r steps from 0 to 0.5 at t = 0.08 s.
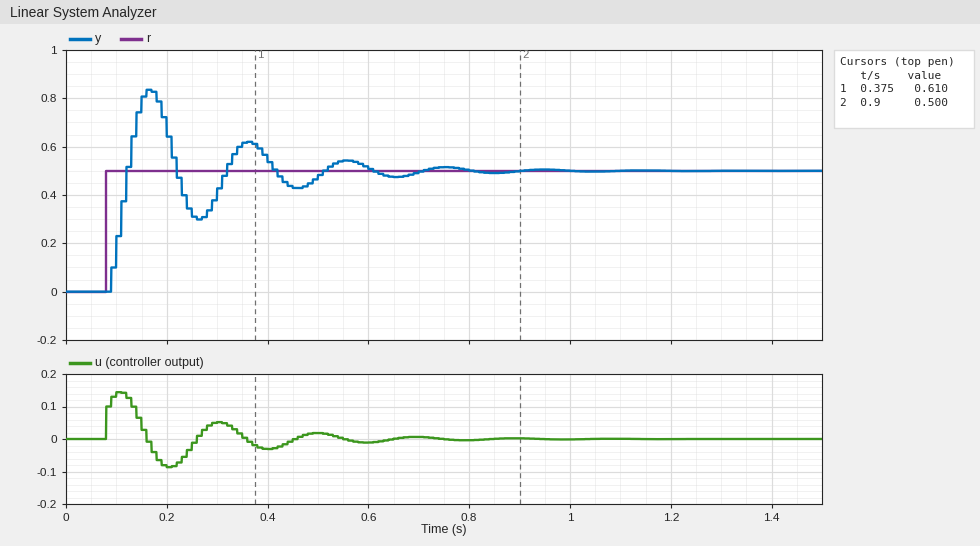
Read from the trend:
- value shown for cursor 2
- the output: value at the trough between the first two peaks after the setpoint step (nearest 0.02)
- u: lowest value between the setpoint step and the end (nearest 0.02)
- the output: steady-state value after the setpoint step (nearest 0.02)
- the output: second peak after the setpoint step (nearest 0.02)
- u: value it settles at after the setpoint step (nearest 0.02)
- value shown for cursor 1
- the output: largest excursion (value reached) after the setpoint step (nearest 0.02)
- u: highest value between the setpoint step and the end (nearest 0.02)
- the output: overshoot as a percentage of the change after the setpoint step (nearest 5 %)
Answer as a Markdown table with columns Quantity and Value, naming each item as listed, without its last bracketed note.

| Quantity | Value |
|---|---|
| value shown for cursor 2 | 0.500 |
| the output: value at the trough between the first two peaks after the setpoint step | 0.30 |
| u: lowest value between the setpoint step and the end | -0.08 |
| the output: steady-state value after the setpoint step | 0.50 |
| the output: second peak after the setpoint step | 0.62 |
| u: value it settles at after the setpoint step | 0.00 |
| value shown for cursor 1 | 0.610 |
| the output: largest excursion (value reached) after the setpoint step | 0.84 |
| u: highest value between the setpoint step and the end | 0.14 |
| the output: overshoot as a percentage of the change after the setpoint step | 65 % |
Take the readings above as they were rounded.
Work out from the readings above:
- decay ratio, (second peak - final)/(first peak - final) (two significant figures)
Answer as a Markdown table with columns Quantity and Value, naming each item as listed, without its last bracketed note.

| Quantity | Value |
|---|---|
| decay ratio, (second peak - final)/(first peak - final) | 0.35 |
